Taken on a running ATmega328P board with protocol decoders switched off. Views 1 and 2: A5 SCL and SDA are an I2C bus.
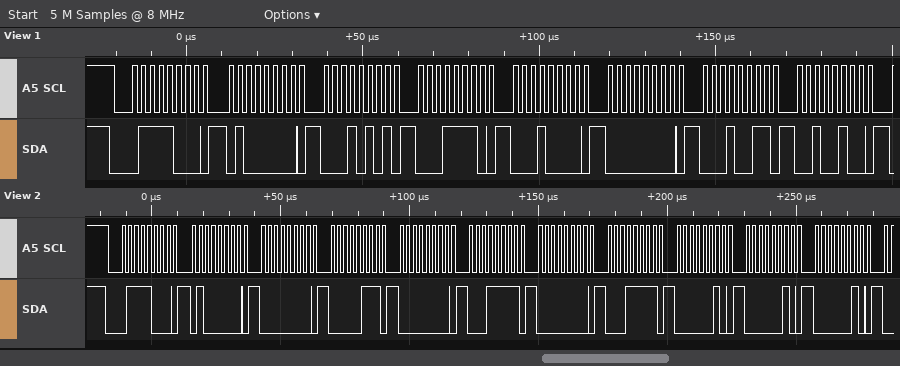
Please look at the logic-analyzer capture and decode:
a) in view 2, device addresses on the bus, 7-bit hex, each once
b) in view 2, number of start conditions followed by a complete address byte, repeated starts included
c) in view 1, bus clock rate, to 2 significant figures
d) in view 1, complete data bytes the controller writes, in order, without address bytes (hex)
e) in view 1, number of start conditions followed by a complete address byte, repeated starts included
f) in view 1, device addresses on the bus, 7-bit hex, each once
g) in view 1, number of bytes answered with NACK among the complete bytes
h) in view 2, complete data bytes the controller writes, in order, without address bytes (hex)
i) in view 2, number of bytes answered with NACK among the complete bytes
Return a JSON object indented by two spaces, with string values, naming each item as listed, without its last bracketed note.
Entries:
{
  "in view 2, device addresses on the bus, 7-bit hex, each once": "0x3C",
  "in view 2, number of start conditions followed by a complete address byte, repeated starts included": "1",
  "in view 1, bus clock rate, to 2 significant figures": "400 kHz",
  "in view 1, complete data bytes the controller writes, in order, without address bytes": "40 15 1E 10 00 13 24",
  "in view 1, number of start conditions followed by a complete address byte, repeated starts included": "1",
  "in view 1, device addresses on the bus, 7-bit hex, each once": "0x3C",
  "in view 1, number of bytes answered with NACK among the complete bytes": "0",
  "in view 2, complete data bytes the controller writes, in order, without address bytes": "40 00 07 00 1F 00 1F 02 02 02",
  "in view 2, number of bytes answered with NACK among the complete bytes": "0"
}
